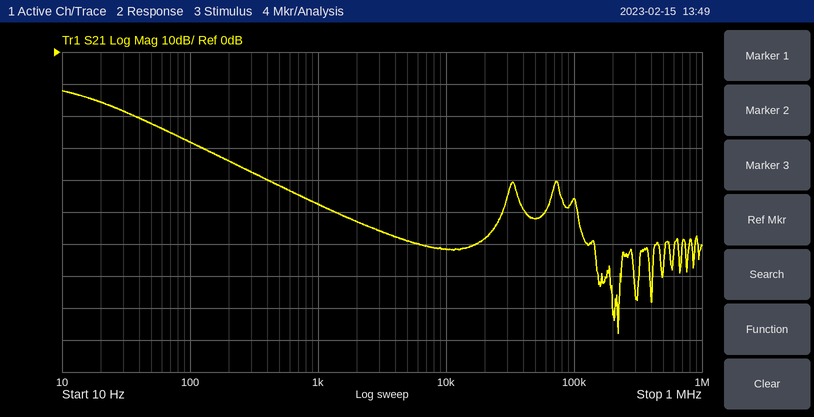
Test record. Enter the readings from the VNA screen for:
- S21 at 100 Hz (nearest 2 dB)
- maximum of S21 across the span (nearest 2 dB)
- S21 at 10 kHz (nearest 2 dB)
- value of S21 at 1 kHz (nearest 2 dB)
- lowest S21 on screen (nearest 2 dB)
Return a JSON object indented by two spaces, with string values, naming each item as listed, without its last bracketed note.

{
  "S21 at 100 Hz": "-28 dB",
  "maximum of S21 across the span": "-12 dB",
  "S21 at 10 kHz": "-62 dB",
  "value of S21 at 1 kHz": "-48 dB",
  "lowest S21 on screen": "-88 dB"
}
